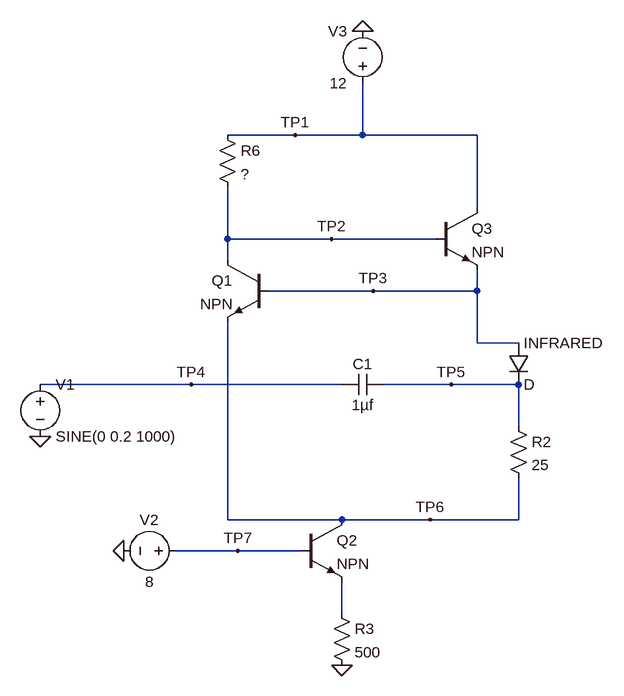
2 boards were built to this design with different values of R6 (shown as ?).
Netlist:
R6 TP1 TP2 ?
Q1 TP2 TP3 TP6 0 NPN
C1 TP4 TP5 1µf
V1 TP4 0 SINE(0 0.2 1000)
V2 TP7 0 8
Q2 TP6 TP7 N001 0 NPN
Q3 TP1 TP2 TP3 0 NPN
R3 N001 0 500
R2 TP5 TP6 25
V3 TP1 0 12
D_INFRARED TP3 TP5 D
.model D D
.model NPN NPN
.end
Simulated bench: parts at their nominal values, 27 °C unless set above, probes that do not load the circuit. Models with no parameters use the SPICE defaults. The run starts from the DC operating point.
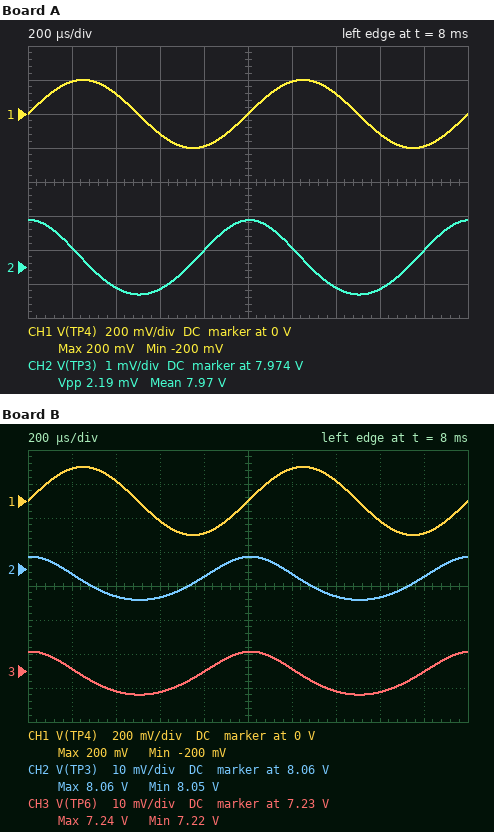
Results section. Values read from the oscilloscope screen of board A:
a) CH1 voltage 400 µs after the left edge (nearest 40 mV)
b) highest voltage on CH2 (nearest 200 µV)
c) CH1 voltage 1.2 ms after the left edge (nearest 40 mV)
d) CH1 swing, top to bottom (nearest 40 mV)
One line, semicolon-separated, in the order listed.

120 mV; 7.9754 V; 200 mV; 400 mV
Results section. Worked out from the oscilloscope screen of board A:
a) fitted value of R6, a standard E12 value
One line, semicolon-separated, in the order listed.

1.2 kΩ
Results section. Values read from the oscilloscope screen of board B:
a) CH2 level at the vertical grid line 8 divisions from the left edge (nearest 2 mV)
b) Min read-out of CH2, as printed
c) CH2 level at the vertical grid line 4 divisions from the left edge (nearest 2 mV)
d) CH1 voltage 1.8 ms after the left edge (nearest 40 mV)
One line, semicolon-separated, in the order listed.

8.052 V; 8.05 V; 8.058 V; -200 mV
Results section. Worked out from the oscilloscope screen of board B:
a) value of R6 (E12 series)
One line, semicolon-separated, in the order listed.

390 Ω
